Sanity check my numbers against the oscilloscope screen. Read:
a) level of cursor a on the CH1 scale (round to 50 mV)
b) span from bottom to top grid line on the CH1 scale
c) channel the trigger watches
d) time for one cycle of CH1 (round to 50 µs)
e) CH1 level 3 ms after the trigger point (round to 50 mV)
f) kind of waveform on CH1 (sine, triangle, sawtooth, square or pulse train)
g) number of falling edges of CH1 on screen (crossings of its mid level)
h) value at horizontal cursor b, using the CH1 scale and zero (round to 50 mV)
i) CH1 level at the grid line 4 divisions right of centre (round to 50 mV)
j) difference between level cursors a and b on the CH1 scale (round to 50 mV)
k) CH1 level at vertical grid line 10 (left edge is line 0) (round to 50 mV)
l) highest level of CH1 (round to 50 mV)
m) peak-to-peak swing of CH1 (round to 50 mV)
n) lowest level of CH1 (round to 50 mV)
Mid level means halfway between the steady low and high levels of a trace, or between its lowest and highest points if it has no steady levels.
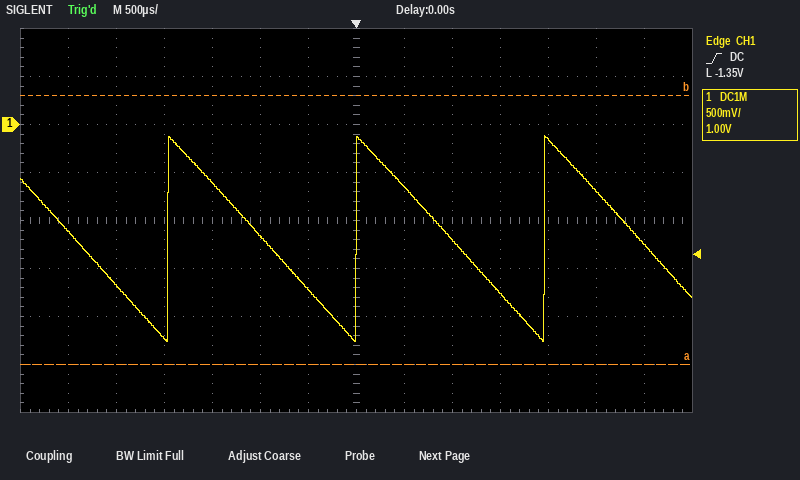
-2.50 V
4 V
CH1
1.95 ms
-1.25 V
sawtooth
4
300 mV
-150 mV
2.80 V
-1.75 V
-100 mV
2.15 V
-2.25 V
